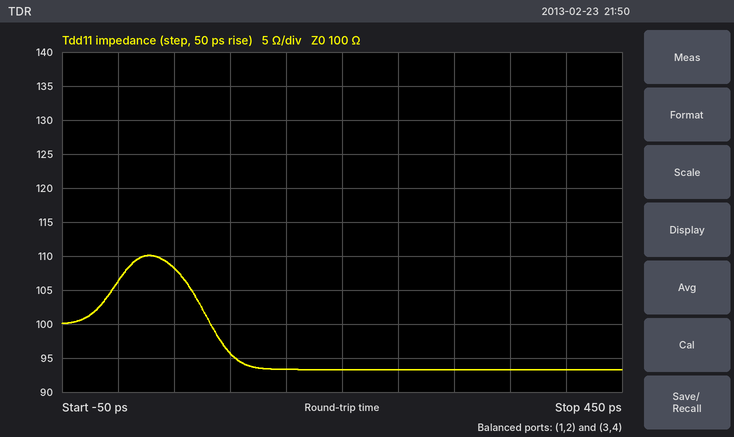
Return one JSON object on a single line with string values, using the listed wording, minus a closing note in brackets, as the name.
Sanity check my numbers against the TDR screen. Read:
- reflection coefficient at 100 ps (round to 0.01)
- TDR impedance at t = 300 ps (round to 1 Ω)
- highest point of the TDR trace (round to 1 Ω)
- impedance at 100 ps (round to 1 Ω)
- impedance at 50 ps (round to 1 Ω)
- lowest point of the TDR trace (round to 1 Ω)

{"reflection coefficient at 100 ps": "-0.02", "TDR impedance at t = 300 ps": "93 Ω", "highest point of the TDR trace": "110 Ω", "impedance at 100 ps": "96 Ω", "impedance at 50 ps": "108 Ω", "lowest point of the TDR trace": "93 Ω"}
